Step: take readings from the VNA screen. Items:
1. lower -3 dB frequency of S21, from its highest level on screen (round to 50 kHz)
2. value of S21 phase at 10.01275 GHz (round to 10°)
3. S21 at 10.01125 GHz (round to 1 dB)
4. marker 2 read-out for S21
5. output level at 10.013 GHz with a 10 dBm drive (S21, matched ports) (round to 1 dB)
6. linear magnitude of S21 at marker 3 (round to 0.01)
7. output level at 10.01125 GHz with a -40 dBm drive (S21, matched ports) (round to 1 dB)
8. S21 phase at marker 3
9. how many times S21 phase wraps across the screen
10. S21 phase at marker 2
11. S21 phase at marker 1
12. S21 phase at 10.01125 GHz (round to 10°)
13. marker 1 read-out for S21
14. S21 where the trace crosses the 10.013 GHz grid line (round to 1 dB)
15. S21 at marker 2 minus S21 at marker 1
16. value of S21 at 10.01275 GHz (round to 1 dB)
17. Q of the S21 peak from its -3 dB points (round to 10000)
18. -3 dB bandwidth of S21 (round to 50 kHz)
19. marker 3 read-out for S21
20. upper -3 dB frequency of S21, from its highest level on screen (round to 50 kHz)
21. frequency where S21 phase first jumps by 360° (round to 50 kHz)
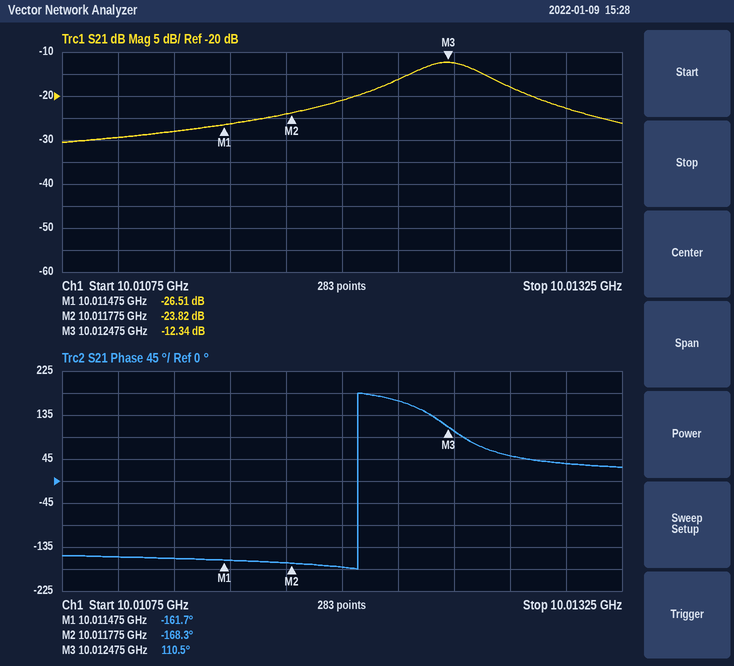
10.01230 GHz
50°
-28 dB
-23.82 dB
-13 dBm
0.24
-68 dBm
110.5°
1
-168.3°
-161.7°
-160°
-26.51 dB
-23 dB
2.69 dB
-18 dB
30000
350 kHz
-12.34 dB
10.01265 GHz
10.01205 GHz
